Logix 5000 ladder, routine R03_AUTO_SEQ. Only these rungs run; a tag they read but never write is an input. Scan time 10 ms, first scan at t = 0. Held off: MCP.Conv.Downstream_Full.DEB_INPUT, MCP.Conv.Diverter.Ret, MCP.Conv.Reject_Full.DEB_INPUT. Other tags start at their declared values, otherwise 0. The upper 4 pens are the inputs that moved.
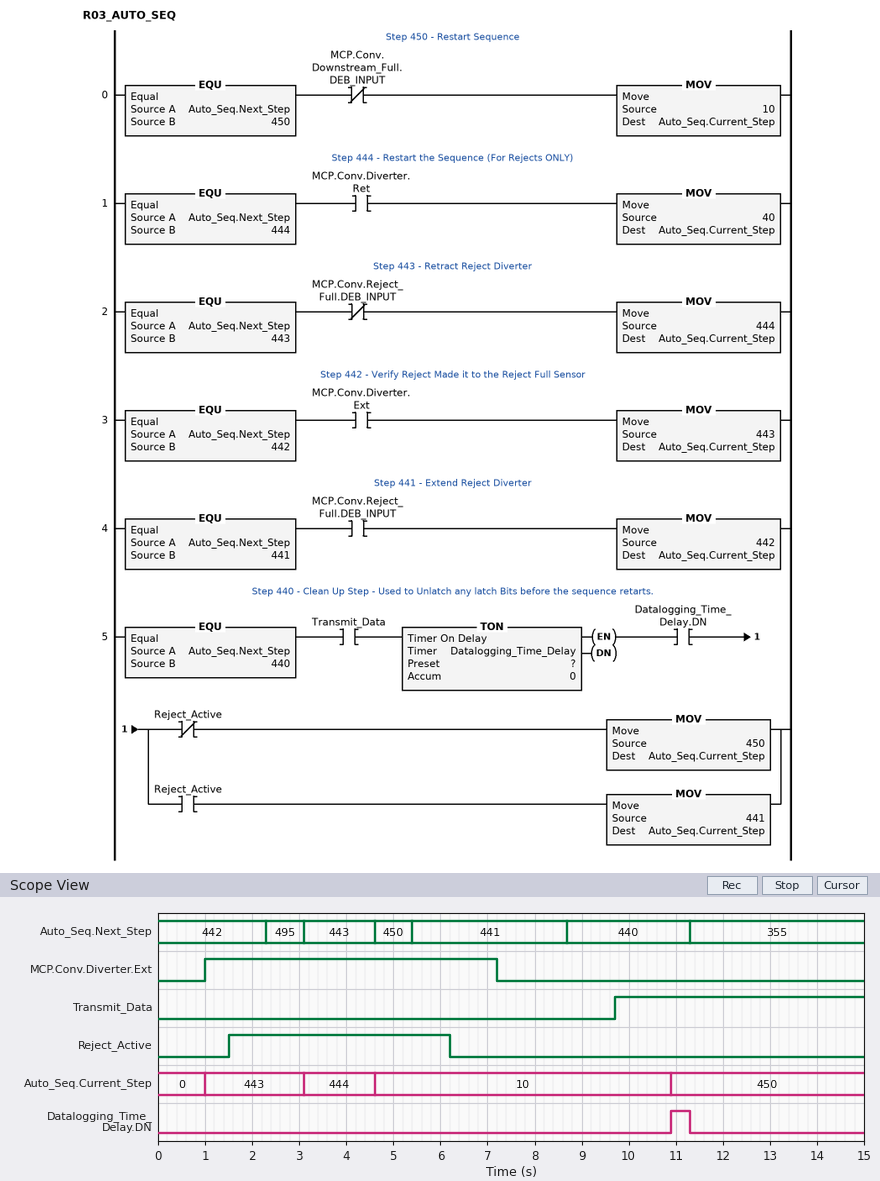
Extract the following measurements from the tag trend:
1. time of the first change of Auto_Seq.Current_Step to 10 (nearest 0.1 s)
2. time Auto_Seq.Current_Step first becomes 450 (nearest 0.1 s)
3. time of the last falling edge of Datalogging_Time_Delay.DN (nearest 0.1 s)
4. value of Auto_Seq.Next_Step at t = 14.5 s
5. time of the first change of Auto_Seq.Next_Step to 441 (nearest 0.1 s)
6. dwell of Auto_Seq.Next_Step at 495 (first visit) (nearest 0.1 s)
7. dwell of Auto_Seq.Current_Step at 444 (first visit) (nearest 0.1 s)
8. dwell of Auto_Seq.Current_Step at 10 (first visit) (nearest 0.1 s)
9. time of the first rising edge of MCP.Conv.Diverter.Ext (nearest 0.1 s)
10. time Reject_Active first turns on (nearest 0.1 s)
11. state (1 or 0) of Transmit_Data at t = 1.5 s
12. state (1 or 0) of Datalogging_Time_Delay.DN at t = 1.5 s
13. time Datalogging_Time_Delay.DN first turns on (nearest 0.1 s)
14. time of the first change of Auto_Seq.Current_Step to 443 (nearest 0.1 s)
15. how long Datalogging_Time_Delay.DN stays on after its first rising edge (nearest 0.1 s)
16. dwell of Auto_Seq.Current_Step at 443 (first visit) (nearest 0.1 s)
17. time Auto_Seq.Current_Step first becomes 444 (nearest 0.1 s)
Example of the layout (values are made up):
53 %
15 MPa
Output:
4.6 s
10.9 s
11.3 s
355
5.4 s
0.8 s
1.5 s
6.3 s
1.0 s
1.5 s
0
0
10.9 s
1.0 s
0.4 s
2.1 s
3.1 s
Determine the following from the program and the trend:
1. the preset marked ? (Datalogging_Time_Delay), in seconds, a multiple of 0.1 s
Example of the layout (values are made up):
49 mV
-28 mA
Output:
1.2 s
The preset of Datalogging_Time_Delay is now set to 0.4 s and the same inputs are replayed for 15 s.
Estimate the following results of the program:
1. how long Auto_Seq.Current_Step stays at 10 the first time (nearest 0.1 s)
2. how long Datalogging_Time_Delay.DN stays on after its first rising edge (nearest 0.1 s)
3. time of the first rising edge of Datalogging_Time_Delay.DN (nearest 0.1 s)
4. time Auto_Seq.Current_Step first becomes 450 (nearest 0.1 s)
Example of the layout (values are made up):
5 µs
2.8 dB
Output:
5.5 s
1.2 s
10.1 s
10.1 s
